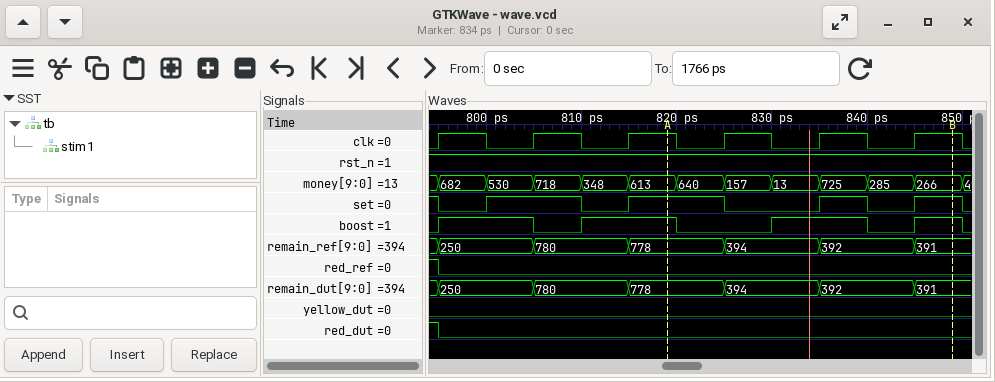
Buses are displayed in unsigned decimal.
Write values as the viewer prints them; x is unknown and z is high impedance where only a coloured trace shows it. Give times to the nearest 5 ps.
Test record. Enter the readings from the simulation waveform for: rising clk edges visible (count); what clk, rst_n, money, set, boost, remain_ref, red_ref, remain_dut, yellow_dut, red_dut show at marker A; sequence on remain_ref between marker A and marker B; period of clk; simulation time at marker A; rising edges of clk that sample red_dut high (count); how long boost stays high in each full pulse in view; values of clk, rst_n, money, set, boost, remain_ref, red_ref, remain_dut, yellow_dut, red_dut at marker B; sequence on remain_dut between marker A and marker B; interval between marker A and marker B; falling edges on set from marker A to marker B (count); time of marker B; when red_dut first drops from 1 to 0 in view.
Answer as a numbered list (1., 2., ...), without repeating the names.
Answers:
1. 6
2. clk=1, rst_n=1, money=613, set=1, boost=1, remain_ref=778, red_ref=0, remain_dut=778, yellow_dut=0, red_dut=0
3. 778, 394, 392, 391
4. 10 ps
5. 820 ps
6. 1
7. 10 ps, 10 ps, 10 ps, 5 ps
8. clk=1, rst_n=1, money=266, set=1, boost=1, remain_ref=391, red_ref=0, remain_dut=391, yellow_dut=0, red_dut=0
9. 778, 394, 392, 391
10. 30 ps
11. 2
12. 850 ps
13. 795 ps
